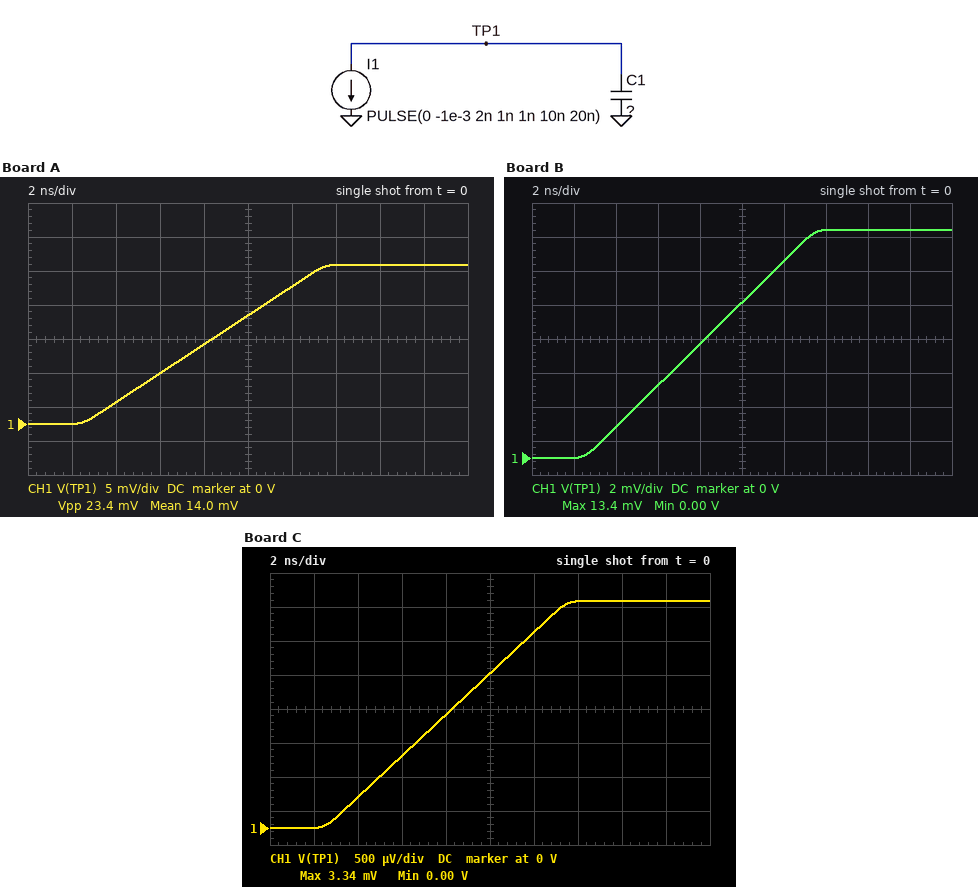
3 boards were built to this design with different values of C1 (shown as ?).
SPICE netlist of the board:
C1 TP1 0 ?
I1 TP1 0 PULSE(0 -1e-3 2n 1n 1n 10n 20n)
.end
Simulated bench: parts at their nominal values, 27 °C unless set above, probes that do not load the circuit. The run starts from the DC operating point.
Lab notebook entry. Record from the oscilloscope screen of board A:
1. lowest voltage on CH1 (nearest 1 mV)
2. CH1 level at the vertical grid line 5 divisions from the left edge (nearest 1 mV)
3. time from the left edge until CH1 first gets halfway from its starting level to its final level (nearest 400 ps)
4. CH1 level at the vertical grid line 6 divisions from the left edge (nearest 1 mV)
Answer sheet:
0 V
16 mV
8.0 ns
20 mV
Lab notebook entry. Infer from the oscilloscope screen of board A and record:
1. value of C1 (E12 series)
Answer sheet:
470 pF
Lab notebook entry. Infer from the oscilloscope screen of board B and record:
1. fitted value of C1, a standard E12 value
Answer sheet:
820 pF
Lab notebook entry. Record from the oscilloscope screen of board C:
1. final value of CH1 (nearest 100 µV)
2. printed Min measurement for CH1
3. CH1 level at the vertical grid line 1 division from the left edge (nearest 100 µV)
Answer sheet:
3.3 mV
0.00 V
0 V
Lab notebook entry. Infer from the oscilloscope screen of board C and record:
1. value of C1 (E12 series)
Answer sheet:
3.3 nF
